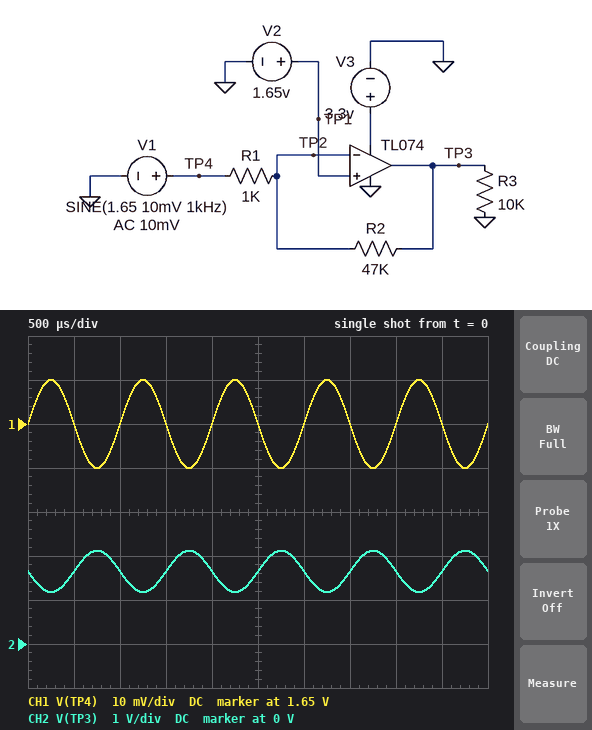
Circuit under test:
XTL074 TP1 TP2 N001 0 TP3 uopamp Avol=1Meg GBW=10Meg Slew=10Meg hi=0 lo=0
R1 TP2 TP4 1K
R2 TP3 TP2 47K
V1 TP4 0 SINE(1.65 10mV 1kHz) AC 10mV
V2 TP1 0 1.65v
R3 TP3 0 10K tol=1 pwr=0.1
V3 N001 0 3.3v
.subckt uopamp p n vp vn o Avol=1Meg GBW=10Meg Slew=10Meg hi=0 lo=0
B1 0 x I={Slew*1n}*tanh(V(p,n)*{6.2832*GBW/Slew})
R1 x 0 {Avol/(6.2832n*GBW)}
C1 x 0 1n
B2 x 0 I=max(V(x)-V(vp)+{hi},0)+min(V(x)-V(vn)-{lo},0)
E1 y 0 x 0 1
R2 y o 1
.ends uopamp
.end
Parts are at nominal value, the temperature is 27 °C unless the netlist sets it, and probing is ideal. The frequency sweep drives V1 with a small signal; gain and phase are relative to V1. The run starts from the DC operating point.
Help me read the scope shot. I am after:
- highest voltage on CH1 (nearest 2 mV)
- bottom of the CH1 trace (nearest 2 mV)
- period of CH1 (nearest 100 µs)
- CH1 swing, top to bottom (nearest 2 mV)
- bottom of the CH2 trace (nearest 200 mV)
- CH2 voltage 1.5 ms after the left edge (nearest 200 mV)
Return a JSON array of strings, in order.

["1.660 V", "1.640 V", "1.0 ms", "20 mV", "1.2 V", "1.6 V"]
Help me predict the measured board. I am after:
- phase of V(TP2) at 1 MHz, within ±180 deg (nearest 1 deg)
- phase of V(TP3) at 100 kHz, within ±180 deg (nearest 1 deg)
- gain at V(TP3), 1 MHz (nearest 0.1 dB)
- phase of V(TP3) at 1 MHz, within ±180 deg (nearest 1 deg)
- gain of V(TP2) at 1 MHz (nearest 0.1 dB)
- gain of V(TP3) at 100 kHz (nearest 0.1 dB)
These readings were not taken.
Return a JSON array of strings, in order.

["12 deg", "154 deg", "19.6 dB", "102 deg", "-0.4 dB", "32.5 dB"]
